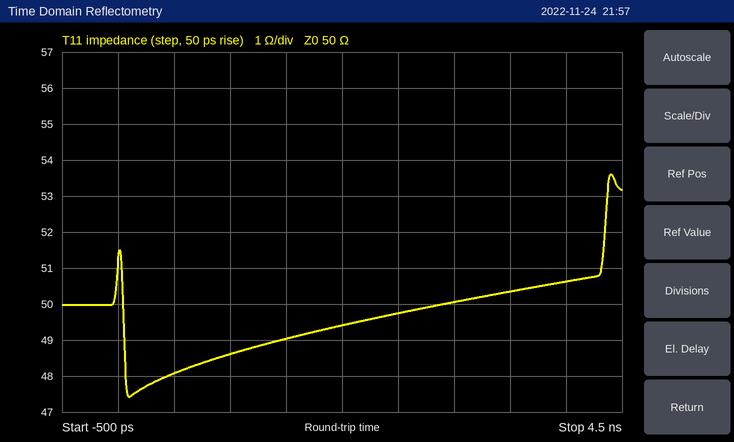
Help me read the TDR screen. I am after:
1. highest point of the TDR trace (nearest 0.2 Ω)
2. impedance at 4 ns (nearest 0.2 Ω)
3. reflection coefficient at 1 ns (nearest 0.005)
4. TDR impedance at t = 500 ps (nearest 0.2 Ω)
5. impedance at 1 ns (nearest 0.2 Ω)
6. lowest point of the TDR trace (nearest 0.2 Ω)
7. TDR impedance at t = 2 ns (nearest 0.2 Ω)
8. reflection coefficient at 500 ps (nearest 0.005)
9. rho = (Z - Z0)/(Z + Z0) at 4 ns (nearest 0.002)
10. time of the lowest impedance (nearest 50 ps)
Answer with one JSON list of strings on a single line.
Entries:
["53.6 Ω", "50.6 Ω", "-0.015", "48.0 Ω", "48.6 Ω", "47.4 Ω", "49.4 Ω", "-0.020", "+0.006", "100 ps"]
